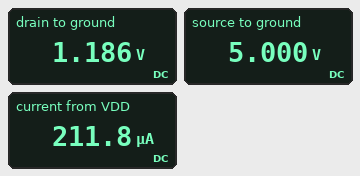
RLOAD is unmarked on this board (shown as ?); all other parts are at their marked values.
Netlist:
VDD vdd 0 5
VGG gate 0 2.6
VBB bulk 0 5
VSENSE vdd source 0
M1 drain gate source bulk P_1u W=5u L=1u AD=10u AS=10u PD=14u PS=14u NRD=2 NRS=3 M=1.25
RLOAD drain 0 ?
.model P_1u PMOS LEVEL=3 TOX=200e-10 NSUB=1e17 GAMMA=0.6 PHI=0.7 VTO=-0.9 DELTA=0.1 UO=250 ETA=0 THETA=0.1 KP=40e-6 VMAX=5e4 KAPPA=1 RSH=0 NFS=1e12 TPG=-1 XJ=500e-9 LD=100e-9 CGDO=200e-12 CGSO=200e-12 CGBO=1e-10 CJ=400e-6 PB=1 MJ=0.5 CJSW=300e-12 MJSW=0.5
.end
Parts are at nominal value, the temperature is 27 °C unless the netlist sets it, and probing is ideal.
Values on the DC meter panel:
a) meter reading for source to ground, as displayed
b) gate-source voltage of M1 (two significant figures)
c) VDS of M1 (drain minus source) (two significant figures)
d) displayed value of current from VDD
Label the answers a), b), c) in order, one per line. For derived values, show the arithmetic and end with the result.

a) 5.000 V
b) 2.6 V - 5 V = -2.4 V
c) 1.186 V - 5 V = -3.8 V
d) 211.8 µA
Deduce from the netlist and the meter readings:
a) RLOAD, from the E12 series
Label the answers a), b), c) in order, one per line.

a) 5.6 kΩ
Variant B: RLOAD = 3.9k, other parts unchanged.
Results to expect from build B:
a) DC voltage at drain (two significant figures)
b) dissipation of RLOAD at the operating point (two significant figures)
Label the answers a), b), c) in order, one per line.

a) 840 mV
b) 180 µW
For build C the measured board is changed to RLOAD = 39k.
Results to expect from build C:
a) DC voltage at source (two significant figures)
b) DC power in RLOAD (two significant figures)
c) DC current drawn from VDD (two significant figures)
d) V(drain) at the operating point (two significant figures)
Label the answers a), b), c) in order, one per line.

a) 5.0 V
b) 540 µW
c) 120 µA
d) 4.6 V
